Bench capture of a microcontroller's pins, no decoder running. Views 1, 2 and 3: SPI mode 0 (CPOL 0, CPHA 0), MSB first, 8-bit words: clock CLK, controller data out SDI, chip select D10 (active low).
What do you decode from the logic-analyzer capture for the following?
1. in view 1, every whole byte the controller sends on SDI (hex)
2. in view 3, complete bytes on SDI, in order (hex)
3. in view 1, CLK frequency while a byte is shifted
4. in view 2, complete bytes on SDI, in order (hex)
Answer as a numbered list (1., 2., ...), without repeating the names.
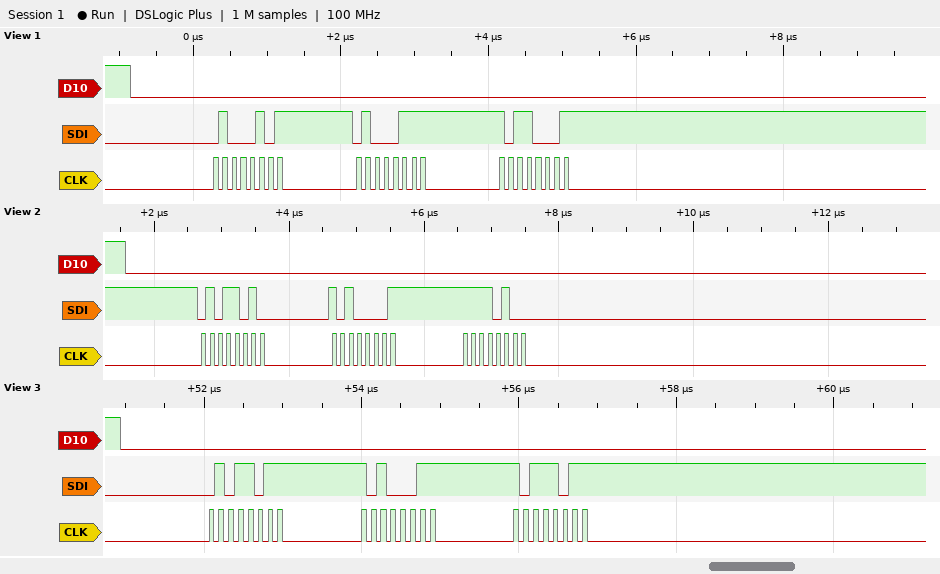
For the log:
1. 0x45 0x47 0xB1
2. 5B A3 BB
3. 8 MHz
4. 5A A1 F4
